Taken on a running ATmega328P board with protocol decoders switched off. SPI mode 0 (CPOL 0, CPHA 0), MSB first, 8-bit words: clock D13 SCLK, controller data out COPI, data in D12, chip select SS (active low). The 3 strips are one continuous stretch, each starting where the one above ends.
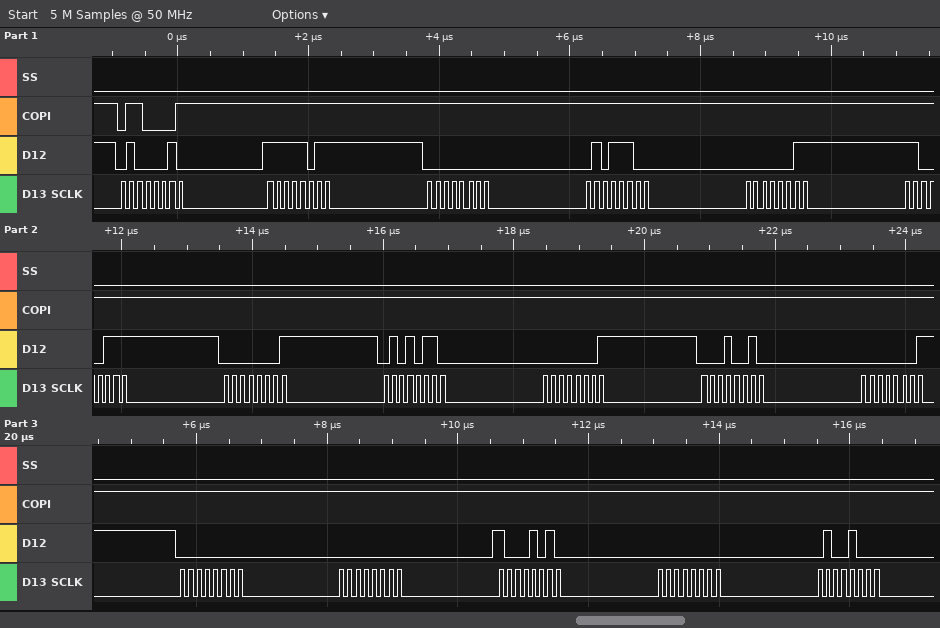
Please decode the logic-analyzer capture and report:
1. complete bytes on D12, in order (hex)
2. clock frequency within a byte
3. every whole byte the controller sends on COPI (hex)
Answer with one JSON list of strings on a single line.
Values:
["42 FB 00 5C 03 C7 01 56 01 12 01 00 00 8A 00 48", "8 MHz", "61 FF FF FF FF FF FF FF FF FF FF FF FF FF FF FF"]
